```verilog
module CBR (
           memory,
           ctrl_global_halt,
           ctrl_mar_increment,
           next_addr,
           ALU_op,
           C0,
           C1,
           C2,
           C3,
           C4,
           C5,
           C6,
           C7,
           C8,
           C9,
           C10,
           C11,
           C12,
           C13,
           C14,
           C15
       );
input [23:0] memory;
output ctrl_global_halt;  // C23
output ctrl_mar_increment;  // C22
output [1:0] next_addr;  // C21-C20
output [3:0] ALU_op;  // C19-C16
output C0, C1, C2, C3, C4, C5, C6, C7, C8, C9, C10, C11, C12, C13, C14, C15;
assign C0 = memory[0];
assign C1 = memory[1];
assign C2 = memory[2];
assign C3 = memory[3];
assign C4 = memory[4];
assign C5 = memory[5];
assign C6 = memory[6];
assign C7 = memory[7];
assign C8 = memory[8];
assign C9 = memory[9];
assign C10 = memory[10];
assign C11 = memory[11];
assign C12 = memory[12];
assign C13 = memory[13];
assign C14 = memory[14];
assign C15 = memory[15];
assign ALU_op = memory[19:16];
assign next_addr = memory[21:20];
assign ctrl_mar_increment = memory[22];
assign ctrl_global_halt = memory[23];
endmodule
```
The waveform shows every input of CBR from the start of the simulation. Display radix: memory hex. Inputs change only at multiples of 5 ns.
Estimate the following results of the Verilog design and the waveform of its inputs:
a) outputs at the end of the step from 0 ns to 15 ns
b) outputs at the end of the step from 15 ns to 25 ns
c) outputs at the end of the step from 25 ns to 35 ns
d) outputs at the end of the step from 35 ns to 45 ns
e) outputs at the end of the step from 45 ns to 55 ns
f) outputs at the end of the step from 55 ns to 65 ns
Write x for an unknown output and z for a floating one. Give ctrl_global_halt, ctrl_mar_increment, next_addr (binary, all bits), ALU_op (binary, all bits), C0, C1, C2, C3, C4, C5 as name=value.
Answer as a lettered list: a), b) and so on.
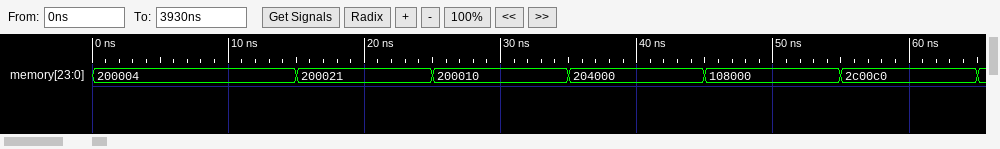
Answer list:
a) ctrl_global_halt=0, ctrl_mar_increment=0, next_addr=10, ALU_op=0000, C0=0, C1=0, C2=1, C3=0, C4=0, C5=0
b) ctrl_global_halt=0, ctrl_mar_increment=0, next_addr=10, ALU_op=0000, C0=1, C1=0, C2=0, C3=0, C4=0, C5=1
c) ctrl_global_halt=0, ctrl_mar_increment=0, next_addr=10, ALU_op=0000, C0=0, C1=0, C2=0, C3=0, C4=1, C5=0
d) ctrl_global_halt=0, ctrl_mar_increment=0, next_addr=10, ALU_op=0000, C0=0, C1=0, C2=0, C3=0, C4=0, C5=0
e) ctrl_global_halt=0, ctrl_mar_increment=0, next_addr=01, ALU_op=0000, C0=0, C1=0, C2=0, C3=0, C4=0, C5=0
f) ctrl_global_halt=0, ctrl_mar_increment=0, next_addr=10, ALU_op=1100, C0=0, C1=0, C2=0, C3=0, C4=0, C5=0
